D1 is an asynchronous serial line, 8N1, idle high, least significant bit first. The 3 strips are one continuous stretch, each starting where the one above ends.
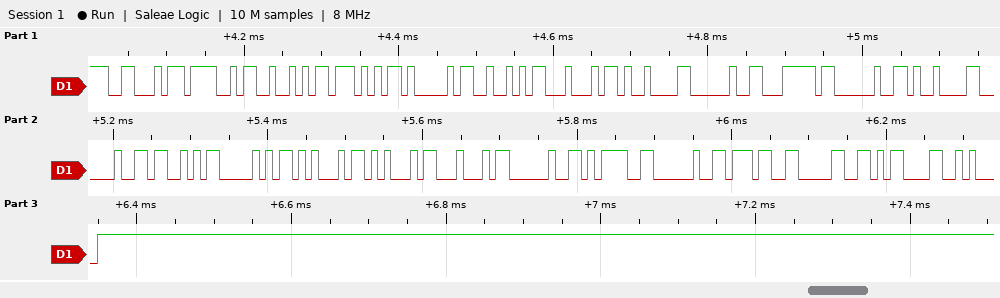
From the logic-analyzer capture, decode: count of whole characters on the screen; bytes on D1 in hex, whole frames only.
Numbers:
25
0x46 0x4F 0x52 0x57 0x41 0x52 0x44 0x09 0x20 0x7C 0x20 0x09 0x20 0x53 0x50 0x45 0x45 0x44 0x20 0x3D 0x20 0x37 0x30 0x0D 0x0A
